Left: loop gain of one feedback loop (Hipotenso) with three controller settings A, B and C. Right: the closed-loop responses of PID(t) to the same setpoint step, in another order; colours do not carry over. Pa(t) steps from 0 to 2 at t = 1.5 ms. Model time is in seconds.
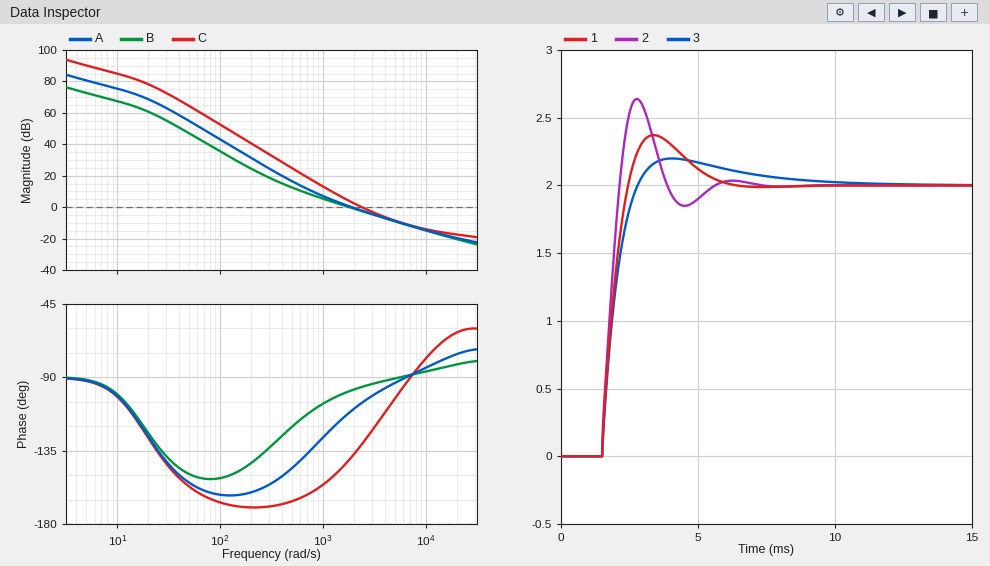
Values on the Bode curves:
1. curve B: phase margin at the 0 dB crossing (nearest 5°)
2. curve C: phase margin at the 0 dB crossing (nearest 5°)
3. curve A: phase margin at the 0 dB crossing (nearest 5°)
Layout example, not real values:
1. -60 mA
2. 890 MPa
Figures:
1. 80°
2. 50°
3. 70°
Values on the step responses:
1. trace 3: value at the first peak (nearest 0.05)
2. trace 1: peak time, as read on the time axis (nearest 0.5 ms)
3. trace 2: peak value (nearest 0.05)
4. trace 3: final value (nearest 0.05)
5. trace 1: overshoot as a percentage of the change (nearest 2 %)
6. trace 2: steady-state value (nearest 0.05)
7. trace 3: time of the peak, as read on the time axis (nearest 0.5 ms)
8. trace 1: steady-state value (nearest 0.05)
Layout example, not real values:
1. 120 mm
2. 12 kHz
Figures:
1. 2.20
2. 3.5 ms
3. 2.65
4. 2.00
5. 18 %
6. 2.00
7. 4.0 ms
8. 2.00
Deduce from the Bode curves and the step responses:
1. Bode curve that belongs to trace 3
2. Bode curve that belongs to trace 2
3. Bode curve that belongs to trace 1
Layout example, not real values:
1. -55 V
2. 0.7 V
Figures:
1. B
2. C
3. A
